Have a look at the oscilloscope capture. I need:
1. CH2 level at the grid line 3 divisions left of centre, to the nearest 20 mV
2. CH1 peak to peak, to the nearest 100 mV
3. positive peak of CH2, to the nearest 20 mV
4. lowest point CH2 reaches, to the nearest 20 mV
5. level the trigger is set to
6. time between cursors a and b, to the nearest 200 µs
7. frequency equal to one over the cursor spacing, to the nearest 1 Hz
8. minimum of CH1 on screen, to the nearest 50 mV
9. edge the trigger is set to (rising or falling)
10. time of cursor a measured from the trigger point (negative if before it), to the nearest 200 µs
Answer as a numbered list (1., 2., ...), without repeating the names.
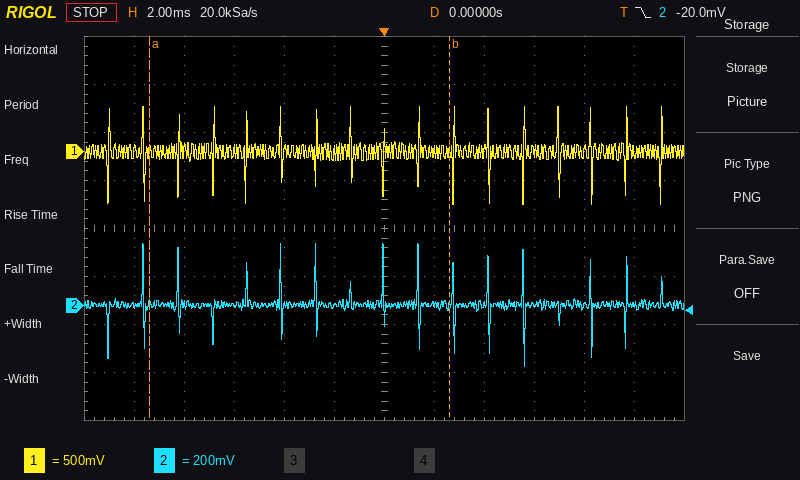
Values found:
1. 0 mV
2. 1.00 V
3. 260 mV
4. -260 mV
5. -20.0 mV
6. 12.0 ms
7. 83 Hz
8. -550 mV
9. falling
10. -9.4 ms
